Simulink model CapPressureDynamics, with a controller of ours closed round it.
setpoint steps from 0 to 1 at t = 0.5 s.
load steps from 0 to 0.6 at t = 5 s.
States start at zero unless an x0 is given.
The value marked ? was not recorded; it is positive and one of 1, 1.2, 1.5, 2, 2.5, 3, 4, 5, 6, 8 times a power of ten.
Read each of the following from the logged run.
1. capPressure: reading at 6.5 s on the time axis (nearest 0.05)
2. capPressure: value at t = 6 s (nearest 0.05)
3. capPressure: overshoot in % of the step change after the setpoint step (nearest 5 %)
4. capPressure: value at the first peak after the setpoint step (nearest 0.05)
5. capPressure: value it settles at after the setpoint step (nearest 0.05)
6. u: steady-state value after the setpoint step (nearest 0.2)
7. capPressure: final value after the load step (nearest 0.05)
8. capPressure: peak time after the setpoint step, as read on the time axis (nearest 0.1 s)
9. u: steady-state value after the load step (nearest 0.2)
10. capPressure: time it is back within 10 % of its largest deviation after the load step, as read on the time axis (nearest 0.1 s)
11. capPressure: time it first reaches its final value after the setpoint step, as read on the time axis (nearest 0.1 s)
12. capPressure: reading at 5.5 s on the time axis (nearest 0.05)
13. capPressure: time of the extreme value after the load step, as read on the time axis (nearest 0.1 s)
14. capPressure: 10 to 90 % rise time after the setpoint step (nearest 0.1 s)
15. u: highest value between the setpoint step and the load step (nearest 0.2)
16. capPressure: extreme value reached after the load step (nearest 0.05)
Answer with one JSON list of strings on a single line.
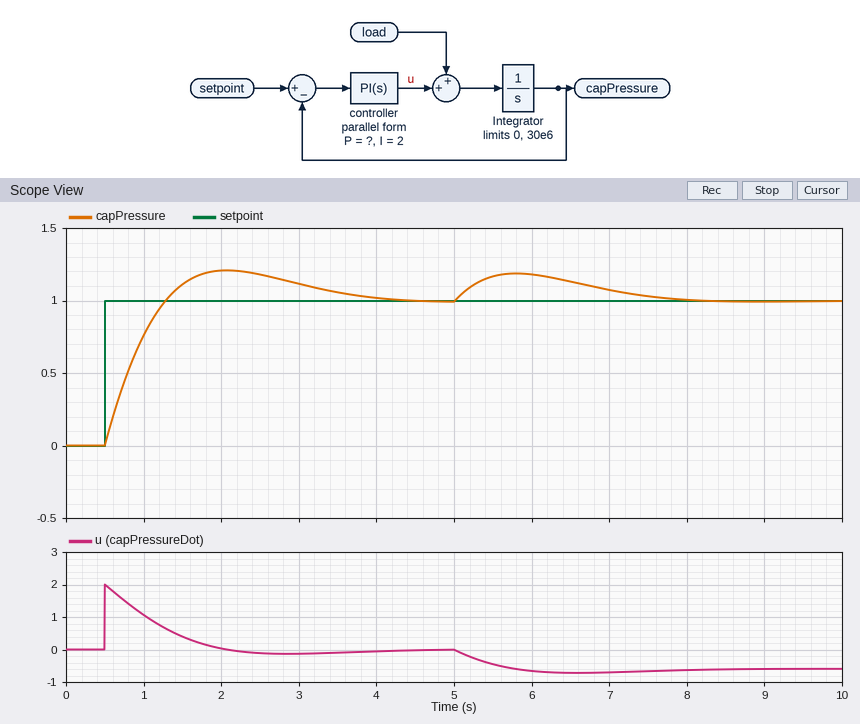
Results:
["1.15", "1.20", "20 %", "1.20", "1.00", "0.0", "1.00", "2.1 s", "-0.6", "7.7 s", "1.3 s", "1.15", "5.8 s", "0.6 s", "2.0", "1.20"]
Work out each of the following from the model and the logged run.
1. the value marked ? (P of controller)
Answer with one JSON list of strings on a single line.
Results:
["2"]
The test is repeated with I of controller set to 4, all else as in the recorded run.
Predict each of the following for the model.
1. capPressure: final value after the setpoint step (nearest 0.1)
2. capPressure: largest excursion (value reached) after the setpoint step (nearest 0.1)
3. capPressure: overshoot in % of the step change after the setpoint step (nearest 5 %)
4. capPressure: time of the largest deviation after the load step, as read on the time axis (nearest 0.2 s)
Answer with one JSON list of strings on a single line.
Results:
["1.0", "1.3", "30 %", "5.6 s"]
